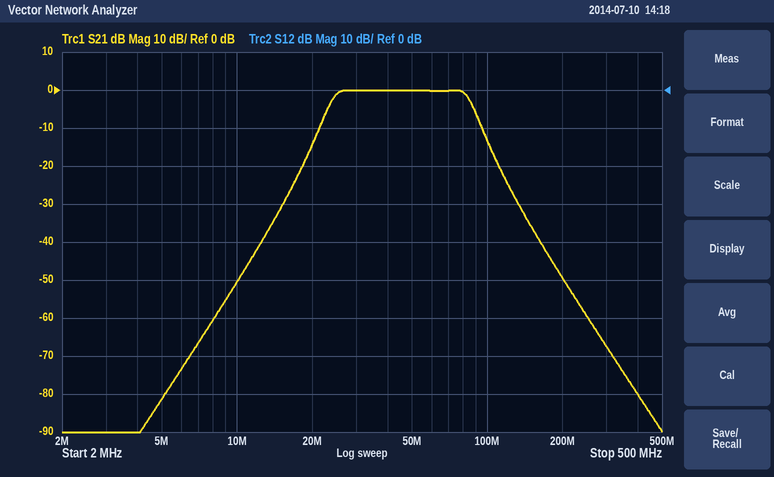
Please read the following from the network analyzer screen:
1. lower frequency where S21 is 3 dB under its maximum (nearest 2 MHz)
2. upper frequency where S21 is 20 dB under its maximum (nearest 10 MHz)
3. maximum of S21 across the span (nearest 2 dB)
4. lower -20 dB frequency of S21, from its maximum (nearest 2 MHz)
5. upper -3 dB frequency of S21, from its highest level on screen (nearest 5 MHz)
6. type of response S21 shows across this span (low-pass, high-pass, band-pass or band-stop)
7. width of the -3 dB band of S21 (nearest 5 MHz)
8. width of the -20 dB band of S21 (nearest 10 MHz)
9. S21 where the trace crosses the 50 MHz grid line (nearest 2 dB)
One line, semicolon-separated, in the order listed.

24 MHz; 110 MHz; 0 dB; 18 MHz; 85 MHz; band-pass; 60 MHz; 90 MHz; 0 dB
